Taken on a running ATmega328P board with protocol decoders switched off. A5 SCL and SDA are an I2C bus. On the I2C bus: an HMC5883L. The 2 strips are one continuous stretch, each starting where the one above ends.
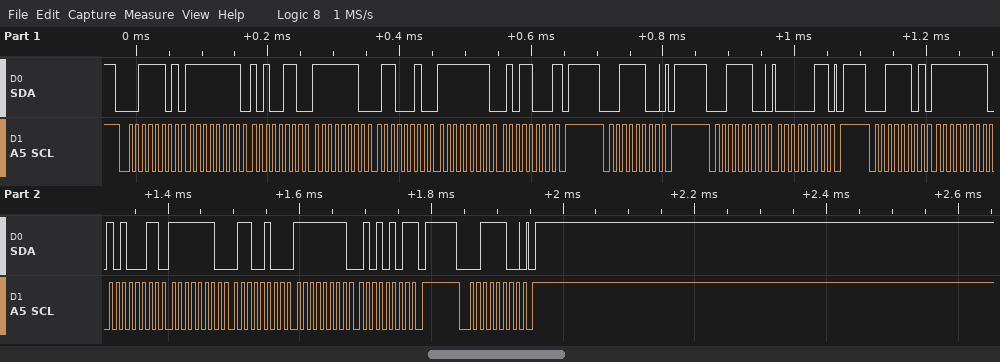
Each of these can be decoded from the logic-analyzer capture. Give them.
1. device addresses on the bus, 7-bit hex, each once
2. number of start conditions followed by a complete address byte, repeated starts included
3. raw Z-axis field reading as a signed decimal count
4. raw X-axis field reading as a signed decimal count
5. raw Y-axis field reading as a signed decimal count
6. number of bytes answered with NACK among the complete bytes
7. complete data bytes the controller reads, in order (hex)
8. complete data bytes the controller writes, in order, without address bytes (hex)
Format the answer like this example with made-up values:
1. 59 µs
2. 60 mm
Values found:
1. 0x1E
2. 5
3. -412
4. -93
5. -171
6. 2
7. FF A6 FE 62 FF 58 FF A3 FE 64 FF 55
8. 03
